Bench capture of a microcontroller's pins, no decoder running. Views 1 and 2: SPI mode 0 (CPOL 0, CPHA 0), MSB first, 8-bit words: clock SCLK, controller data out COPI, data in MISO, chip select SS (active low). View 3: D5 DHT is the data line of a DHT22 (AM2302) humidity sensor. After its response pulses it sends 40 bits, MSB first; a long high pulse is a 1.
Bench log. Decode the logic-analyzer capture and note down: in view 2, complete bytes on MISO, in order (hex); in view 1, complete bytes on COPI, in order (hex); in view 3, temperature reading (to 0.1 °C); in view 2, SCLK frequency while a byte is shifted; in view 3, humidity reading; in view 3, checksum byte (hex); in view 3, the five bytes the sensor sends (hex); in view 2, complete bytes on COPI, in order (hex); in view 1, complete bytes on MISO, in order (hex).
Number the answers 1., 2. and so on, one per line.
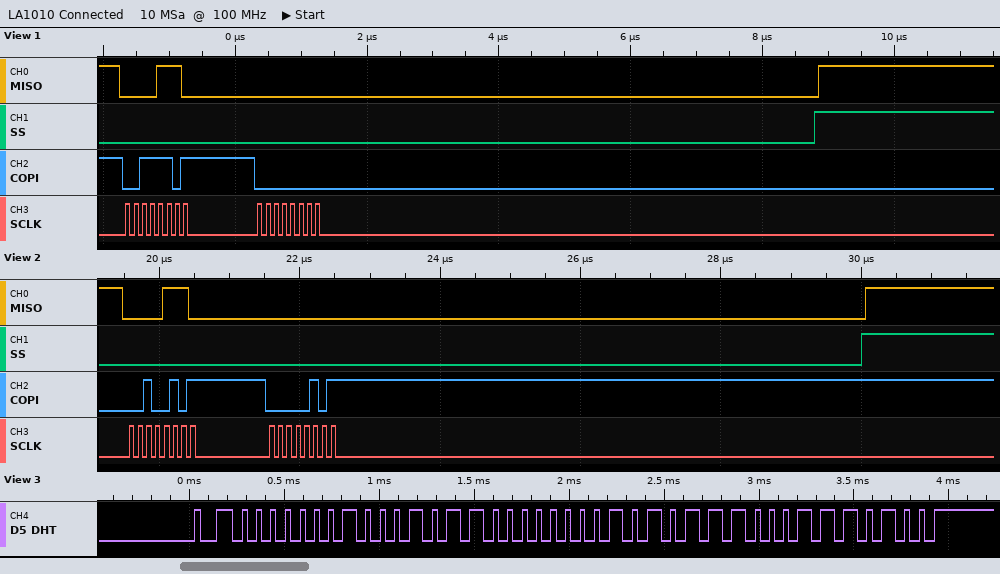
1. 0E 00
2. 0x3D 0x00
3. 34.8 °C
4. 8 MHz
5. 27.8 %
6. 0x74
7. 01 16 01 5C 74
8. 25 05
9. 0x0E 0x00
